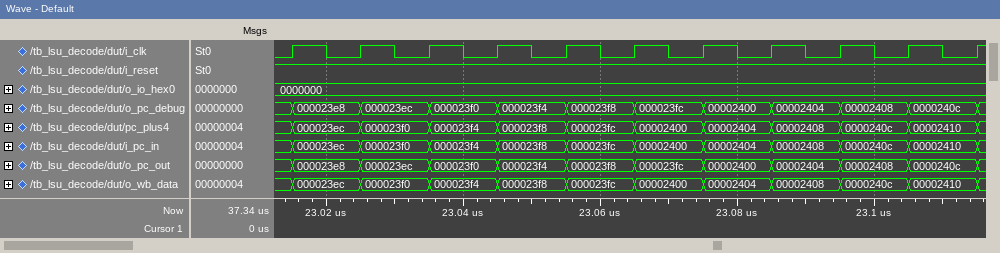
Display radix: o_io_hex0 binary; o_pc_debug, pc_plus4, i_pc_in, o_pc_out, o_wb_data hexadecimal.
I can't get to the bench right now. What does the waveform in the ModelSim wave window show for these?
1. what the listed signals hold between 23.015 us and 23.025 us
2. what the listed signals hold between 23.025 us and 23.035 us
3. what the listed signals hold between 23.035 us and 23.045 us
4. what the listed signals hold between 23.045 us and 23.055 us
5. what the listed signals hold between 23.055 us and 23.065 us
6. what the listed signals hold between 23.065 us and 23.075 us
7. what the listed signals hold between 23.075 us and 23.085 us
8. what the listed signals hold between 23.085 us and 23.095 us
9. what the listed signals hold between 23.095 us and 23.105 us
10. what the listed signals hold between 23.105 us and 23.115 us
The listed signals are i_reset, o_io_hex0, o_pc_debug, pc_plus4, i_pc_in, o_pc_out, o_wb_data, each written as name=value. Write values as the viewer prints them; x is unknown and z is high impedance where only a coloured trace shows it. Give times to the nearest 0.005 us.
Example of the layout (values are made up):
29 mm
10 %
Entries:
i_reset=1, o_io_hex0=0000000, o_pc_debug=000023e8, pc_plus4=000023ec, i_pc_in=000023ec, o_pc_out=000023e8, o_wb_data=000023ec
i_reset=1, o_io_hex0=0000000, o_pc_debug=000023ec, pc_plus4=000023f0, i_pc_in=000023f0, o_pc_out=000023ec, o_wb_data=000023f0
i_reset=1, o_io_hex0=0000000, o_pc_debug=000023f0, pc_plus4=000023f4, i_pc_in=000023f4, o_pc_out=000023f0, o_wb_data=000023f4
i_reset=1, o_io_hex0=0000000, o_pc_debug=000023f4, pc_plus4=000023f8, i_pc_in=000023f8, o_pc_out=000023f4, o_wb_data=000023f8
i_reset=1, o_io_hex0=0000000, o_pc_debug=000023f8, pc_plus4=000023fc, i_pc_in=000023fc, o_pc_out=000023f8, o_wb_data=000023fc
i_reset=1, o_io_hex0=0000000, o_pc_debug=000023fc, pc_plus4=00002400, i_pc_in=00002400, o_pc_out=000023fc, o_wb_data=00002400
i_reset=1, o_io_hex0=0000000, o_pc_debug=00002400, pc_plus4=00002404, i_pc_in=00002404, o_pc_out=00002400, o_wb_data=00002404
i_reset=1, o_io_hex0=0000000, o_pc_debug=00002404, pc_plus4=00002408, i_pc_in=00002408, o_pc_out=00002404, o_wb_data=00002408
i_reset=1, o_io_hex0=0000000, o_pc_debug=00002408, pc_plus4=0000240c, i_pc_in=0000240c, o_pc_out=00002408, o_wb_data=0000240c
i_reset=1, o_io_hex0=0000000, o_pc_debug=0000240c, pc_plus4=00002410, i_pc_in=00002410, o_pc_out=0000240c, o_wb_data=00002410
